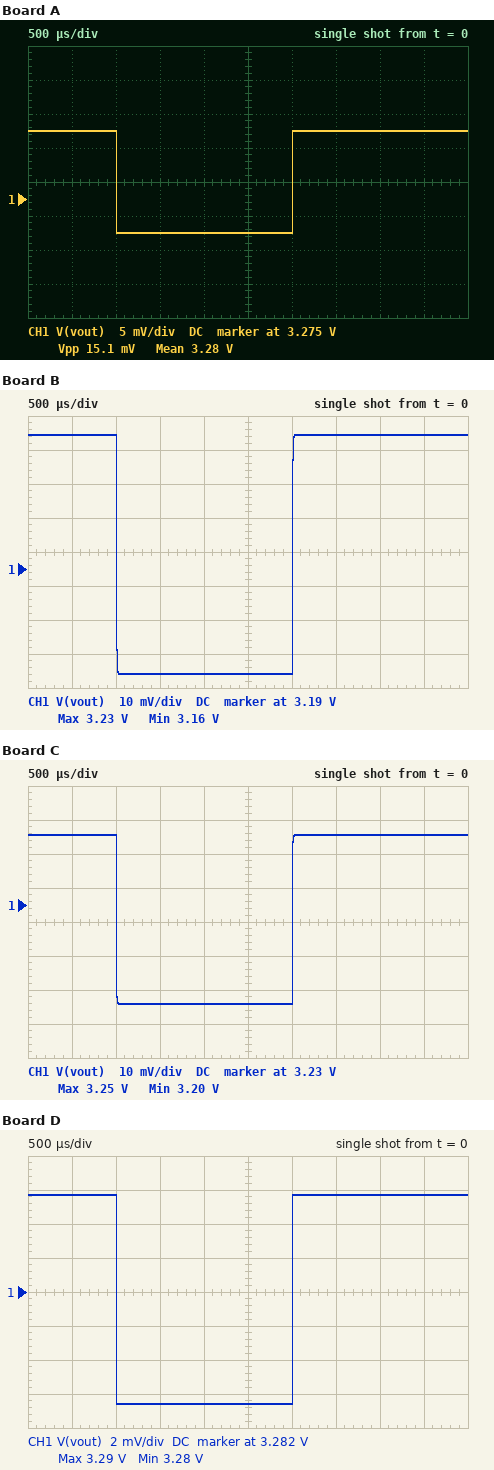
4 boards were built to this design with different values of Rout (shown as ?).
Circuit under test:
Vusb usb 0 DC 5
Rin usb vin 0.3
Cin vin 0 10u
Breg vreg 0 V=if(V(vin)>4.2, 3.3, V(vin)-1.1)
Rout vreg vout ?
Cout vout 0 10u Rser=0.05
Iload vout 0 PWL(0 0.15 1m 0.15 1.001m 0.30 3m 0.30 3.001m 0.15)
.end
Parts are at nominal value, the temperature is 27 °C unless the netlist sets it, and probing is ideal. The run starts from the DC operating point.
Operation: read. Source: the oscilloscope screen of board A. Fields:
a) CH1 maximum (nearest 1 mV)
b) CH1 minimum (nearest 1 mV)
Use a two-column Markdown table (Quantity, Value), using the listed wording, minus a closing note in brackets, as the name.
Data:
| Quantity | Value |
|---|---|
| CH1 maximum | 3.285 V |
| CH1 minimum | 3.270 V |
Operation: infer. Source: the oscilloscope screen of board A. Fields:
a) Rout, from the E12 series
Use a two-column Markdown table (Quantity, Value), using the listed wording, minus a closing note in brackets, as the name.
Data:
| Quantity | Value |
|---|---|
| Rout, from the E12 series | 0.1 Ω |
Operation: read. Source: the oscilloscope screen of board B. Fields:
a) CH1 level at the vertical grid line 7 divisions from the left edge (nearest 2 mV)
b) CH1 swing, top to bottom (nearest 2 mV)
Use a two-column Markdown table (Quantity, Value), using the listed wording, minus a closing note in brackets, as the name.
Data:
| Quantity | Value |
|---|---|
| CH1 level at the vertical grid line 7 divisions from the left edge | 3.230 V |
| CH1 swing, top to bottom | 70 mV |
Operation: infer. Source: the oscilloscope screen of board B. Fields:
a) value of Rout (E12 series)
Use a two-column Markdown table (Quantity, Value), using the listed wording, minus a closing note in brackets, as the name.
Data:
| Quantity | Value |
|---|---|
| value of Rout | 0.47 Ω |
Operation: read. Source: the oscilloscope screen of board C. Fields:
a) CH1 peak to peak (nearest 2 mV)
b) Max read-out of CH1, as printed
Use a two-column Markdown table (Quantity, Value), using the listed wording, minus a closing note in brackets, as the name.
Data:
| Quantity | Value |
|---|---|
| CH1 peak to peak | 50 mV |
| Max read-out of CH1, as printed | 3.25 V |
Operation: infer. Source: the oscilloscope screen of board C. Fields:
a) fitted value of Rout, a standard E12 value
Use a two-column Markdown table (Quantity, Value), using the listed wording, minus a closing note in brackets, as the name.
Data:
| Quantity | Value |
|---|---|
| fitted value of Rout, a standard E12 value | 0.33 Ω |
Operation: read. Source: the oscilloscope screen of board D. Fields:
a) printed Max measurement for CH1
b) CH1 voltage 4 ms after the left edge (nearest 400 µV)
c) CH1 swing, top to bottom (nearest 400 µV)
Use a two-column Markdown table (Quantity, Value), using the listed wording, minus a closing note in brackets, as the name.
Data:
| Quantity | Value |
|---|---|
| printed Max measurement for CH1 | 3.29 V |
| CH1 voltage 4 ms after the left edge | 3.2876 V |
| CH1 swing, top to bottom | 12.4 mV |
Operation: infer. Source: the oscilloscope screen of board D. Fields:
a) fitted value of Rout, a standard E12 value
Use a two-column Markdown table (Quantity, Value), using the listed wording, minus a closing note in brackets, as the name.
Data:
| Quantity | Value |
|---|---|
| fitted value of Rout, a standard E12 value | 0.082 Ω |
